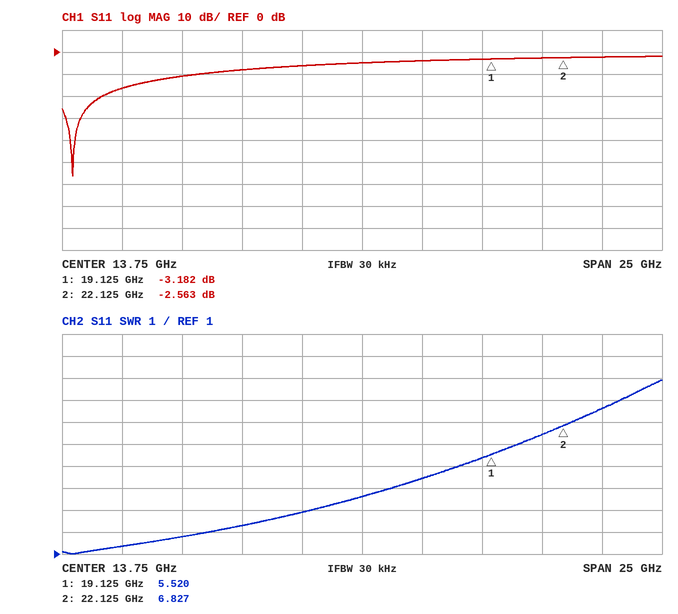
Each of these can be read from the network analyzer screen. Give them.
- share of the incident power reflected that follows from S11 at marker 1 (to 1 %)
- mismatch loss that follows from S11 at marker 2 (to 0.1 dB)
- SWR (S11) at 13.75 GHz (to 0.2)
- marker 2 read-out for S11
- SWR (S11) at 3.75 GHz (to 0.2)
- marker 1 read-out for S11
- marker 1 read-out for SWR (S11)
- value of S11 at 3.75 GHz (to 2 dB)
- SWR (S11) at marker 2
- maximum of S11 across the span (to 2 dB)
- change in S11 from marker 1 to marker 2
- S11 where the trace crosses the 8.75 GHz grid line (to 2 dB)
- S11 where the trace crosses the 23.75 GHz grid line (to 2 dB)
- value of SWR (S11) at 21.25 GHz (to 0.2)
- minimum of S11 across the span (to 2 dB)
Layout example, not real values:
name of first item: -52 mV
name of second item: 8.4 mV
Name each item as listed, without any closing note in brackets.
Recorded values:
share of the incident power reflected that follows from S11 at marker 1: 48 %
mismatch loss that follows from S11 at marker 2: 3.5 dB
SWR (S11) at 13.75 GHz: 3.6
marker 2 read-out for S11: -2.563 dB
SWR (S11) at 3.75 GHz: 1.4
marker 1 read-out for S11: -3.182 dB
marker 1 read-out for SWR: 5.520
value of S11 at 3.75 GHz: -16 dB
SWR (S11) at marker 2: 6.827
maximum of S11 across the span: -2 dB
change in S11 from marker 1 to marker 2: 0.619 dB
S11 where the trace crosses the 8.75 GHz grid line: -8 dB
S11 where the trace crosses the 23.75 GHz grid line: -2 dB
value of SWR (S11) at 21.25 GHz: 6.4
minimum of S11 across the span: -56 dB
